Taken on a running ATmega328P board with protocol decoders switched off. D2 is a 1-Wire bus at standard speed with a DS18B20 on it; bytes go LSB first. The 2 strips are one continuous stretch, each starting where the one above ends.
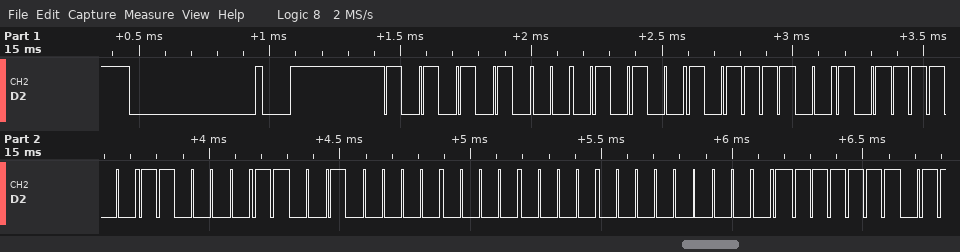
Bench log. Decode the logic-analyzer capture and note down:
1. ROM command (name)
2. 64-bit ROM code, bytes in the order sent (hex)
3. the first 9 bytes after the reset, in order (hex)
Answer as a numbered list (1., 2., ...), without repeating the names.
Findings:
1. Match ROM
2. 28 3D 3D C3 04 00 00 FE
3. 55 28 3D 3D C3 04 00 00 FE
